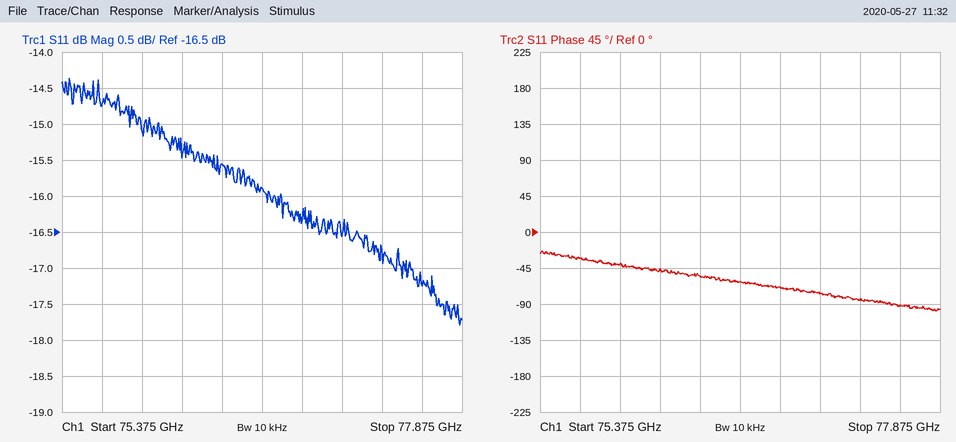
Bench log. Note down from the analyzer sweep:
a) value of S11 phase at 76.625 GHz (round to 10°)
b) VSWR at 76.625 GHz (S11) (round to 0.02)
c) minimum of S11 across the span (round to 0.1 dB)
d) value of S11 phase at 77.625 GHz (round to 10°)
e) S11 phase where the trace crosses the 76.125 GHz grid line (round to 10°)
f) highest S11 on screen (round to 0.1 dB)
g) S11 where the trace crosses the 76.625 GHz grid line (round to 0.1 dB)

-60°
1.38
-17.8 dB
-90°
-50°
-14.4 dB
-15.9 dB
